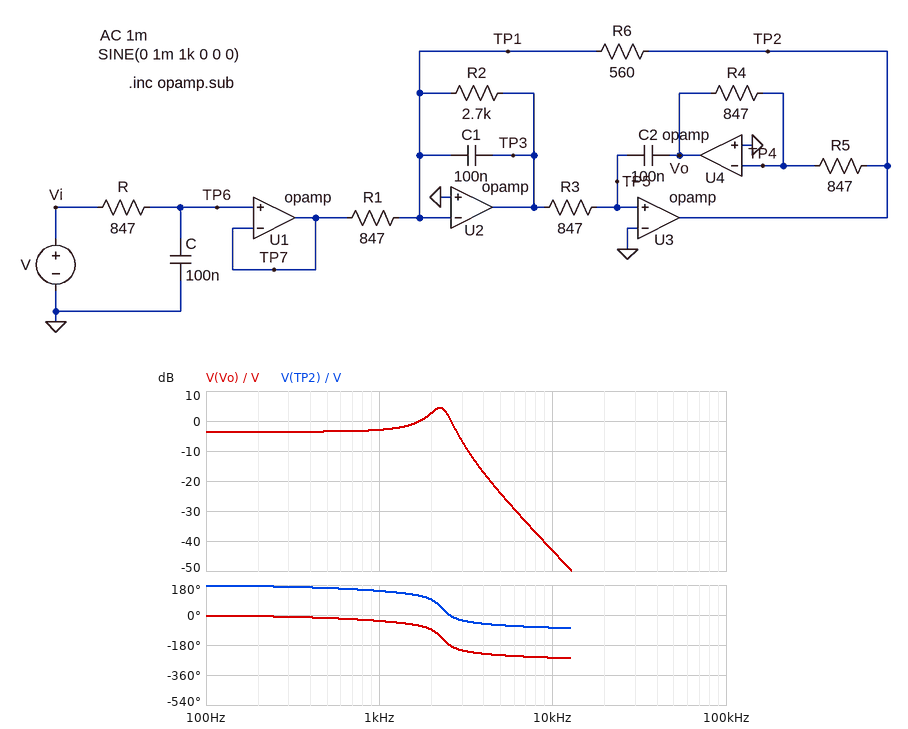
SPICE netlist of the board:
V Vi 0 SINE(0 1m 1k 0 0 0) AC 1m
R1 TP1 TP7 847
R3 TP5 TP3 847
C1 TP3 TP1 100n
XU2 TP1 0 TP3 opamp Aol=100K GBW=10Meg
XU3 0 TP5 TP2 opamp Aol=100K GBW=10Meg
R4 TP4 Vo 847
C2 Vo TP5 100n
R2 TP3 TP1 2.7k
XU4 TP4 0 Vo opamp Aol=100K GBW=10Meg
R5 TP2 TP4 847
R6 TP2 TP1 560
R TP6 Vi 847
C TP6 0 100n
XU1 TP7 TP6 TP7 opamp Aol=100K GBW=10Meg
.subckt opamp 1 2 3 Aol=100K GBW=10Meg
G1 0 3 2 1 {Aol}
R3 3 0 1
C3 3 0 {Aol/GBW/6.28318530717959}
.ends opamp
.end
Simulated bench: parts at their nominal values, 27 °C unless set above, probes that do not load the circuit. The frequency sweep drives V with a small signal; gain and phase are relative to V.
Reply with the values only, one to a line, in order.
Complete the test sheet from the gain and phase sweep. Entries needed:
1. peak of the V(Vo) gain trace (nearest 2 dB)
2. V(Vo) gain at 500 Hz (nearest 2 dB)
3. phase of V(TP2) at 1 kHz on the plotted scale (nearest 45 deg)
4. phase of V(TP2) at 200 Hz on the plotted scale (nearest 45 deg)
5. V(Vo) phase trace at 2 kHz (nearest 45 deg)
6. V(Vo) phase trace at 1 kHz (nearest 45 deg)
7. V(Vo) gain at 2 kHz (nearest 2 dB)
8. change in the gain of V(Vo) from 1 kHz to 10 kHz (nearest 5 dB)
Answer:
4 dB
-4 dB
135 deg
180 deg
-90 deg
-45 deg
2 dB
-40 dB
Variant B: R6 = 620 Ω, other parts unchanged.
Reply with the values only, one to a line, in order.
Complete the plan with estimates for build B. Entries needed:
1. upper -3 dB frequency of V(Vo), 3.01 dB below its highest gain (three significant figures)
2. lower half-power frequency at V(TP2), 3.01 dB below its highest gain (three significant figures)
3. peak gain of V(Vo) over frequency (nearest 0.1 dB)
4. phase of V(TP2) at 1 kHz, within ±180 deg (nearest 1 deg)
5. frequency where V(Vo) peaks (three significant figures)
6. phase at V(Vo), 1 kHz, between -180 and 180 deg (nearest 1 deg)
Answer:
2.40 kHz
1.76 kHz
5.2 dB
143 deg
2.13 kHz
-37 deg
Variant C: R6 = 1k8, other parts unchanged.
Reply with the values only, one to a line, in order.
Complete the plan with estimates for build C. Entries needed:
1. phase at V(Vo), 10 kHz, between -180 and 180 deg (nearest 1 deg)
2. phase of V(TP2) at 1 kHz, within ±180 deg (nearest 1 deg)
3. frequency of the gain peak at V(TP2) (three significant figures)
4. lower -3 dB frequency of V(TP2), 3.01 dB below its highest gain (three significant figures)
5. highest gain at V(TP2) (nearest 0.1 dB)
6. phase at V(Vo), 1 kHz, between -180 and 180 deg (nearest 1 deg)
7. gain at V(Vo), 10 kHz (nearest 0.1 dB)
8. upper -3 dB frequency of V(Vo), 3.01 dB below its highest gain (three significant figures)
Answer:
104 deg
110 deg
1.20 kHz
780 Hz
12.1 dB
-70 deg
-43.6 dB
1.46 kHz
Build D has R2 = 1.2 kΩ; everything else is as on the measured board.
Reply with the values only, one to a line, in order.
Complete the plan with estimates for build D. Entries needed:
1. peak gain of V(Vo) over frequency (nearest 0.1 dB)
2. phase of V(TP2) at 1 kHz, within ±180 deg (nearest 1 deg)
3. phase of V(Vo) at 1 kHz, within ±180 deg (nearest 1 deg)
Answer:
-1.8 dB
135 deg
-45 deg
